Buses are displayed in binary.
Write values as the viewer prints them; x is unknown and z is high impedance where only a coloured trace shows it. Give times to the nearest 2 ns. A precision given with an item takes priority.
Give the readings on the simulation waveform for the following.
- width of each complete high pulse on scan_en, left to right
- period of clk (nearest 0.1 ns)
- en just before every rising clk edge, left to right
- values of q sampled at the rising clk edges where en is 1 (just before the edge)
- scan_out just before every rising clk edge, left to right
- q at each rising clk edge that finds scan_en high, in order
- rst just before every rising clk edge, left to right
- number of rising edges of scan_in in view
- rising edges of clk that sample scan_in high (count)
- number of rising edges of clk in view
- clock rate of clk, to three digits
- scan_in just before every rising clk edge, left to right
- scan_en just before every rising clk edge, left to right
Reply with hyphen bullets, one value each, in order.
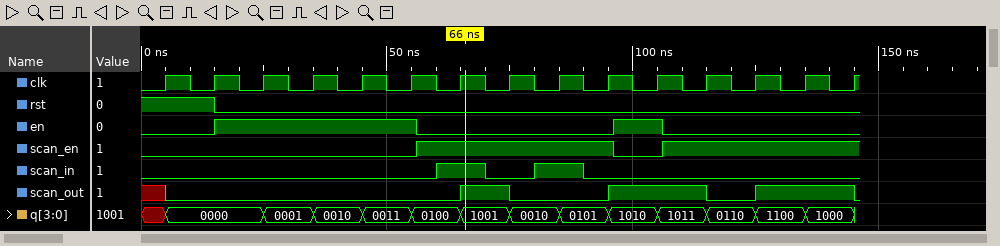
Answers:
- 40 ns
- 10 ns
- 0 0 1 1 1 1 0 0 0 0 1 0 0 0 0
- 0000, 0001, 0010, 0011, 1010
- x 0 0 0 0 0 0 1 0 0 1 1 0 1 1
- 0100, 1001, 0010, 0101, 1011, 0110, 1100, 1000
- 1 1 0 0 0 0 0 0 0 0 0 0 0 0 0
- 2
- 2
- 15
- 100 MHz
- 0 0 0 0 0 0 1 0 1 0 0 0 0 0 0
- 0 0 0 0 0 0 1 1 1 1 0 1 1 1 1
